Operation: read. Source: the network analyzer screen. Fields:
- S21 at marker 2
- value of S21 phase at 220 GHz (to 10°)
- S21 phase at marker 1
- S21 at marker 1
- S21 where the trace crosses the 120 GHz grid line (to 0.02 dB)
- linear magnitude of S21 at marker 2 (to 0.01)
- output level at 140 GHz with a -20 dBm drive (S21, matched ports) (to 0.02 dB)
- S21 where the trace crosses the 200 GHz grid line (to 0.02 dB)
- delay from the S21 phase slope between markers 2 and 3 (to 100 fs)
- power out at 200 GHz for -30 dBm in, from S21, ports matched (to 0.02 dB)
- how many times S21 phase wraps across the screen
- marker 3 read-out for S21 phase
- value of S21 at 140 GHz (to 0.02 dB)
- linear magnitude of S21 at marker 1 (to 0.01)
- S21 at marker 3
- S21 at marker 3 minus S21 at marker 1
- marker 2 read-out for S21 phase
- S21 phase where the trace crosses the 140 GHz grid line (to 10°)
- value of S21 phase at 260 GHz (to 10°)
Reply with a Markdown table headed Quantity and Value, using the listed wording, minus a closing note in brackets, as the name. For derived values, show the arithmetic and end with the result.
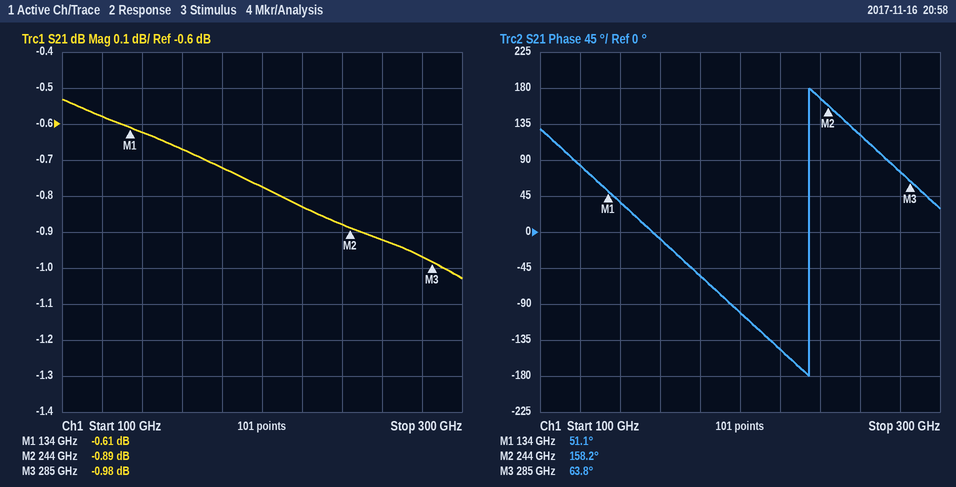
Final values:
| Quantity | Value |
|---|---|
| S21 at marker 2 | -0.89 dB |
| value of S21 phase at 220 GHz | -150° |
| S21 phase at marker 1 | 51.1° |
| S21 at marker 1 | -0.61 dB |
| S21 where the trace crosses the 120 GHz grid line | -0.58 dB |
| linear magnitude of S21 at marker 2 | 10^(-0.89/20) ≈ 0.90 |
| output level at 140 GHz with a -20 dBm drive (S21, matched ports) | -20 dBm + (-0.62 dB) = -20.62 dBm |
| S21 where the trace crosses the 200 GHz grid line | -0.78 dB |
| delay from the S21 phase slope between markers 2 and 3 | −(63.8° − (158.2°))/(360° × 41 GHz) ≈ 6.4 ps |
| power out at 200 GHz for -30 dBm in, from S21, ports matched | -30 dBm + (-0.78 dB) = -30.78 dBm |
| how many times S21 phase wraps across the screen | 1 |
| marker 3 read-out for S21 phase | 63.8° |
| value of S21 at 140 GHz | -0.62 dB |
| linear magnitude of S21 at marker 1 | 10^(-0.61/20) ≈ 0.93 |
| S21 at marker 3 | -0.98 dB |
| S21 at marker 3 minus S21 at marker 1 | -0.98 − (-0.61) = -0.37 dB |
| marker 2 read-out for S21 phase | 158.2° |
| S21 phase where the trace crosses the 140 GHz grid line | 40° |
| value of S21 phase at 260 GHz | 120° |
